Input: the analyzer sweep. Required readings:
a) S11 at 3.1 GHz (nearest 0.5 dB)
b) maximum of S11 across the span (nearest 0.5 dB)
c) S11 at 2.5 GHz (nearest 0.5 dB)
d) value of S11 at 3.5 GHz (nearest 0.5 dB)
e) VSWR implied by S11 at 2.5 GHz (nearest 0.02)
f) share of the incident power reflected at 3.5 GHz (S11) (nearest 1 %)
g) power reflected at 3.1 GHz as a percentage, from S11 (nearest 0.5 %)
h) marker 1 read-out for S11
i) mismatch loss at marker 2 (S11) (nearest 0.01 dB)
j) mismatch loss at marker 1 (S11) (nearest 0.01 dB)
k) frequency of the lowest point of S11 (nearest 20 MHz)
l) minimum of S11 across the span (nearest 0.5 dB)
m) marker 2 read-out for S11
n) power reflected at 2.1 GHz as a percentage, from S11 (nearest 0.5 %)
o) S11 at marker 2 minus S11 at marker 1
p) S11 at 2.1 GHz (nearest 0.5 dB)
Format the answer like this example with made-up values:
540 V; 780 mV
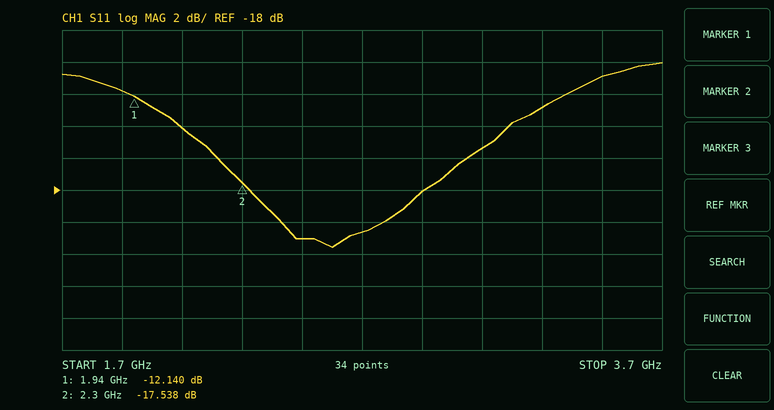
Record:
-15.5 dB; -10.0 dB; -21.0 dB; -11.0 dB; 1.20; 8 %; 3.0 %; -12.140 dB; 0.08 dB; 0.27 dB; 2.60 GHz; -21.5 dB; -17.538 dB; 4.0 %; -5.398 dB; -14.0 dB
